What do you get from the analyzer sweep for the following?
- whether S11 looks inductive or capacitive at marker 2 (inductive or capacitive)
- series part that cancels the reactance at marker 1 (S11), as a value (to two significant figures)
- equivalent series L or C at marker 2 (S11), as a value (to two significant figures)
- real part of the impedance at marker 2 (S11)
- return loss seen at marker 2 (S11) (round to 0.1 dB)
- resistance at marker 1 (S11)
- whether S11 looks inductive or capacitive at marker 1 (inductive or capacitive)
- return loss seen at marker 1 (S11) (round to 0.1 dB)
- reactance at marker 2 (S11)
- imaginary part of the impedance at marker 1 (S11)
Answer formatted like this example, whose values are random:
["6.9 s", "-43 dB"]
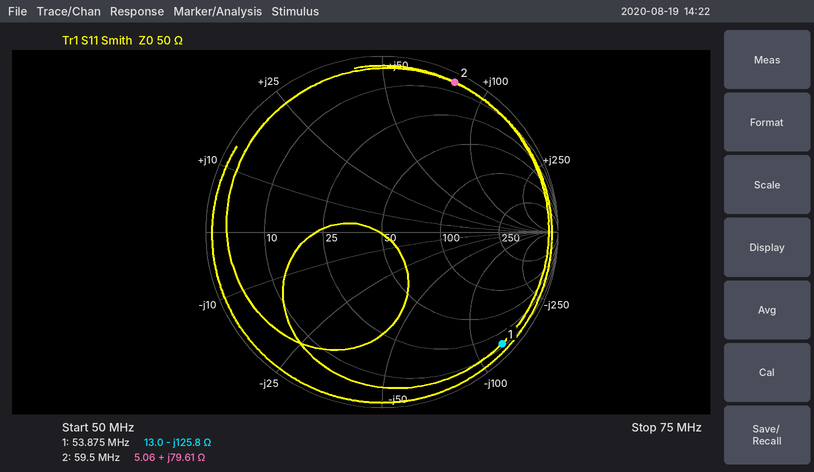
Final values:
["inductive", "370 nH", "210 nH", "5.06 Ω", "0.5 dB", "13.0 Ω", "capacitive", "0.6 dB", "+79.61 Ω", "-125.8 Ω"]
